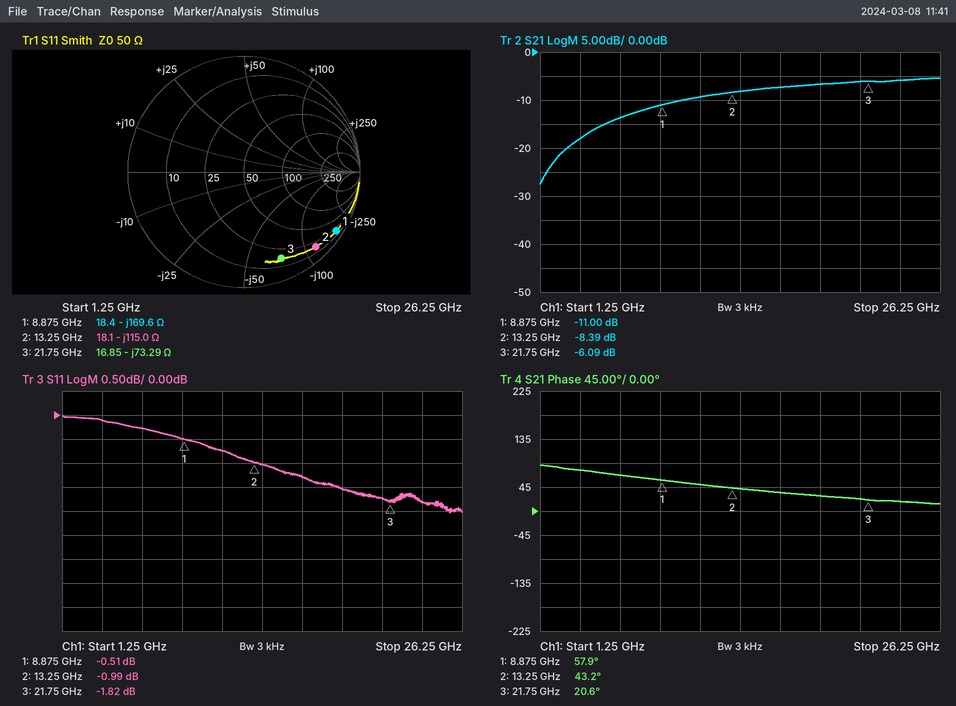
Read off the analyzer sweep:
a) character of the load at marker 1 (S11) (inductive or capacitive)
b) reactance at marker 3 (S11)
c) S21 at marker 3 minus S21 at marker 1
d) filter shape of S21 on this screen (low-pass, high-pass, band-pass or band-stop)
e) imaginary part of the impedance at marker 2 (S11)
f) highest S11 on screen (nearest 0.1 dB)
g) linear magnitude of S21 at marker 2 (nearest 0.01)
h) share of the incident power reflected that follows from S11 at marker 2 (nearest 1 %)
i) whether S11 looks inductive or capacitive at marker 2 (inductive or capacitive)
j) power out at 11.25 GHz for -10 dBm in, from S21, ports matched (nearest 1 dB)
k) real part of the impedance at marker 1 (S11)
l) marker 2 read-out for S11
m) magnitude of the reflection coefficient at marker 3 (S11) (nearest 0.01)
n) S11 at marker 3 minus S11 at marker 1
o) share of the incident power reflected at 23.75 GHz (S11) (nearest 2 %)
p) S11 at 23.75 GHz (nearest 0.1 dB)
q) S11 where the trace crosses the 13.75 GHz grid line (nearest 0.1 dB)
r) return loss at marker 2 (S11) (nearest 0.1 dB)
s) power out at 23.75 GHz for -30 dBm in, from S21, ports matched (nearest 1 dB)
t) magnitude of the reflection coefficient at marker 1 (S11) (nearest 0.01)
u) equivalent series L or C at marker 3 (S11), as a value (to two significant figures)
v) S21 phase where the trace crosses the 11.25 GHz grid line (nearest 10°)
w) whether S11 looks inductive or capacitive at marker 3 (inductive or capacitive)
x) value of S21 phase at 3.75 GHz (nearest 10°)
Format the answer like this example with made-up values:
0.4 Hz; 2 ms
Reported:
capacitive; -73.29 Ω; 4.91 dB; high-pass; -115.0 Ω; 0.0 dB; 0.38; 80 %; capacitive; -19 dBm; 18.4 Ω; -0.99 dB; 0.81; -1.31 dB; 66 %; -1.8 dB; -1.0 dB; 1.0 dB; -36 dBm; 0.94; 100 fF; 50°; capacitive; 80°
